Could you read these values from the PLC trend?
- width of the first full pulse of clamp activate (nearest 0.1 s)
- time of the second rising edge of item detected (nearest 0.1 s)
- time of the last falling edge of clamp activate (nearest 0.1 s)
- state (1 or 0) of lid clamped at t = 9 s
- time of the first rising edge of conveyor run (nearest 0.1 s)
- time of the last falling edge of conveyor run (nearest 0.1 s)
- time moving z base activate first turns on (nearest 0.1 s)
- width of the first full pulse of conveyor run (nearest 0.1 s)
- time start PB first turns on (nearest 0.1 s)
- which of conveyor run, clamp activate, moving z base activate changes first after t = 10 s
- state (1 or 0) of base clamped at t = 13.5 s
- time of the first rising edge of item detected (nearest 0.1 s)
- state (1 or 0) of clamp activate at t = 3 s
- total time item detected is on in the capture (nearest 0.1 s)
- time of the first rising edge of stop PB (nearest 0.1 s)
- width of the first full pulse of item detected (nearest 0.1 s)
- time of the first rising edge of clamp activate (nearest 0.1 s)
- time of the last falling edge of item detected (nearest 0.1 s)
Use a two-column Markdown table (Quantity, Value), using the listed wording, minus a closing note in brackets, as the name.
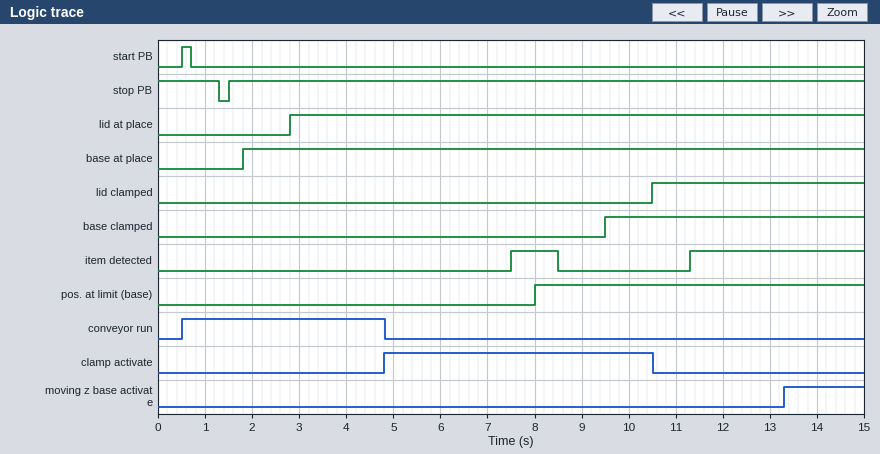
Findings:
| Quantity | Value |
|---|---|
| width of the first full pulse of clamp activate | 5.7 s |
| time of the second rising edge of item detected | 11.3 s |
| time of the last falling edge of clamp activate | 10.5 s |
| state (1 or 0) of lid clamped at t = 9 s | 0 |
| time of the first rising edge of conveyor run | 0.5 s |
| time of the last falling edge of conveyor run | 4.8 s |
| time moving z base activate first turns on | 13.3 s |
| width of the first full pulse of conveyor run | 4.3 s |
| time start PB first turns on | 0.5 s |
| which of conveyor run, clamp activate, moving z base activate changes first after t = 10 s | clamp activate |
| state (1 or 0) of base clamped at t = 13.5 s | 1 |
| time of the first rising edge of item detected | 7.5 s |
| state (1 or 0) of clamp activate at t = 3 s | 0 |
| total time item detected is on in the capture | 4.7 s |
| time of the first rising edge of stop PB | 1.5 s |
| width of the first full pulse of item detected | 1.0 s |
| time of the first rising edge of clamp activate | 4.8 s |
| time of the last falling edge of item detected | 8.5 s |
